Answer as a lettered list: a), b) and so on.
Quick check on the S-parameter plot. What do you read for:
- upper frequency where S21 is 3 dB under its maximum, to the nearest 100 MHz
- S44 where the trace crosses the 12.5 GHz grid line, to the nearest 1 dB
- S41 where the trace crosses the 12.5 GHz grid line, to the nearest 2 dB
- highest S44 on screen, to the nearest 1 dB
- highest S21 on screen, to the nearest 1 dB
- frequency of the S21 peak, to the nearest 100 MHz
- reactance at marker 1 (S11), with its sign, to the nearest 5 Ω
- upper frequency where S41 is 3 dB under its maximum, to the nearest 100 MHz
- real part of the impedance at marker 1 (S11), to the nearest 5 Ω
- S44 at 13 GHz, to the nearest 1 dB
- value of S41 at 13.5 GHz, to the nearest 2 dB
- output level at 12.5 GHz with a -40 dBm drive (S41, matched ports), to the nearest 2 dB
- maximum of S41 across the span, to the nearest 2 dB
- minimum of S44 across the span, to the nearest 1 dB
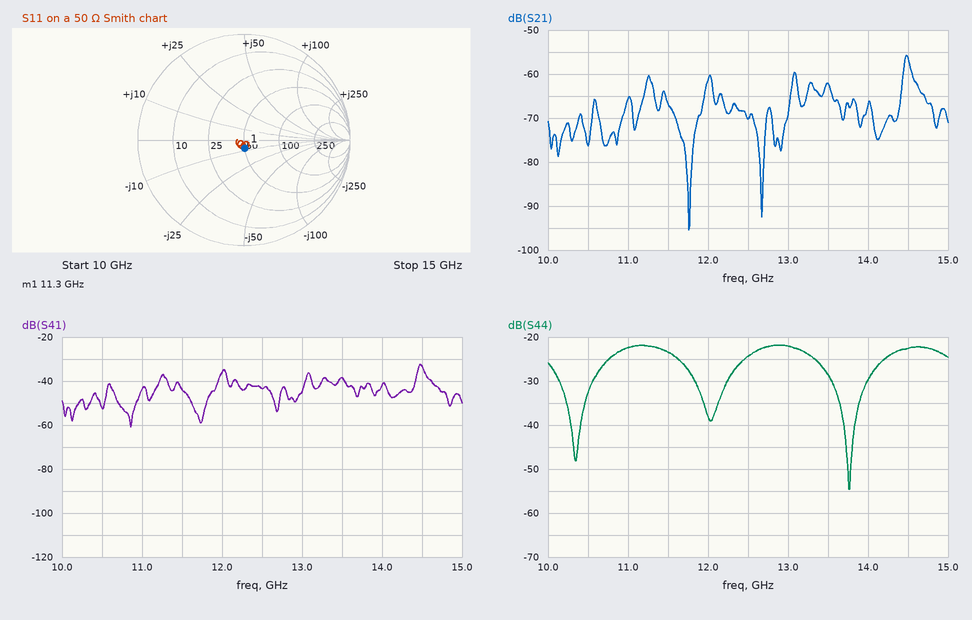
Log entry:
a) 14.5 GHz
b) -24 dB
c) -44 dB
d) -22 dB
e) -56 dB
f) 14.5 GHz
g) -10 Ω
h) 14.5 GHz
i) 50 Ω
j) -22 dB
k) -38 dB
l) -84 dBm
m) -32 dB
n) -55 dB
